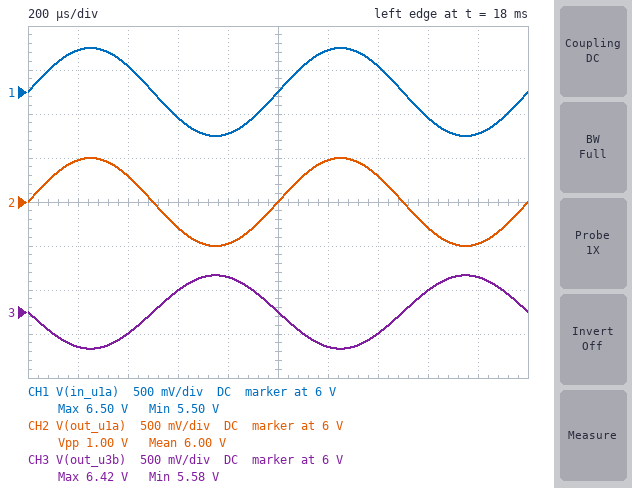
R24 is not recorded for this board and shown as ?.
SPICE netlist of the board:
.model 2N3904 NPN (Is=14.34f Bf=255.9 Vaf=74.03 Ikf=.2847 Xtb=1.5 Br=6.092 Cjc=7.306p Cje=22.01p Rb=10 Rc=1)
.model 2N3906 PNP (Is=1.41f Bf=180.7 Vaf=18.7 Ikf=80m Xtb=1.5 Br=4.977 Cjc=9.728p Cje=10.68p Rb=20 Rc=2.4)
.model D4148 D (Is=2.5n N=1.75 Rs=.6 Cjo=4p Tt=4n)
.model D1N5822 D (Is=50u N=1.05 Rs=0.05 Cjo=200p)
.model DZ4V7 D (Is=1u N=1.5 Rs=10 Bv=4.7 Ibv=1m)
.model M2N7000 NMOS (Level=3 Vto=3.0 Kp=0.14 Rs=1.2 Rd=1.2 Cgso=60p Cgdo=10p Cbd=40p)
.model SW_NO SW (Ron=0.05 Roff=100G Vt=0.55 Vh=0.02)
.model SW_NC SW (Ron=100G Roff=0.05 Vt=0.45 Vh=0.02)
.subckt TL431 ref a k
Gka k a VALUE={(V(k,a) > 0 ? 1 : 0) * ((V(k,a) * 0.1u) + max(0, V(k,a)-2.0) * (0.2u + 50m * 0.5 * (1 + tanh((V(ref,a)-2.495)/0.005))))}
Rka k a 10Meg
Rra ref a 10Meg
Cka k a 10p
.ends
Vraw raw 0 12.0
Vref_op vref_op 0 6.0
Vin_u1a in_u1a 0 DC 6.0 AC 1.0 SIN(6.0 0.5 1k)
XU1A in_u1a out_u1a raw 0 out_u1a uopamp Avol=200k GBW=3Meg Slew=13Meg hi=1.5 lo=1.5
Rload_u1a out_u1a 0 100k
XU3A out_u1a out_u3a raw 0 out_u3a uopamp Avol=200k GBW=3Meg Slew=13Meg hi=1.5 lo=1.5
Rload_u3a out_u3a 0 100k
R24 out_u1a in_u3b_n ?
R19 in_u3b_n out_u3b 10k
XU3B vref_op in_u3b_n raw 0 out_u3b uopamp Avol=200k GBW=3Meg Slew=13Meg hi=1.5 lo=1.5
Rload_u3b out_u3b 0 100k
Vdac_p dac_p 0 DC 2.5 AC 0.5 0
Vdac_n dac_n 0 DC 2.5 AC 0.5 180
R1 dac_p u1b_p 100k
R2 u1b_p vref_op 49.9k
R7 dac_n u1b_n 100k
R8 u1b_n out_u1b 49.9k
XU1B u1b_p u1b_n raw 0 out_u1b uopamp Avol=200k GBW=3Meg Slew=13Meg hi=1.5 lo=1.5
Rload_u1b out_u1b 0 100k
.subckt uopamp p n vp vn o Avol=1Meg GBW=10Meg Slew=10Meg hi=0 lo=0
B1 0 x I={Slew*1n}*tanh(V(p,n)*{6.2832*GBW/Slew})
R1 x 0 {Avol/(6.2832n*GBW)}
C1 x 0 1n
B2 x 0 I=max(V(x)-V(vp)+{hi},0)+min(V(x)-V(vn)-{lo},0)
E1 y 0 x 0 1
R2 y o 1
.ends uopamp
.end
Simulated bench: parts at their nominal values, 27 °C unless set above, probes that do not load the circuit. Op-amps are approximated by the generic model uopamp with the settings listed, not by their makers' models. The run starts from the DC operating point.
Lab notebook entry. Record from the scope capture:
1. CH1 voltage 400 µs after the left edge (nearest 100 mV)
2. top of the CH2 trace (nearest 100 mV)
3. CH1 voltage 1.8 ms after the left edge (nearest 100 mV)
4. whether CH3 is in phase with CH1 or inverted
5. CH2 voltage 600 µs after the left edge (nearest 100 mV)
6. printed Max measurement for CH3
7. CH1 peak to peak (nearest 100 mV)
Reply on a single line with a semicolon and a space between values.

6.3 V; 6.5 V; 5.5 V; inverted; 5.7 V; 6.42 V; 1.0 V
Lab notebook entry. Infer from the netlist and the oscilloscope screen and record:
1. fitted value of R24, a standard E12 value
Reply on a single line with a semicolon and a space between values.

12 kΩ
